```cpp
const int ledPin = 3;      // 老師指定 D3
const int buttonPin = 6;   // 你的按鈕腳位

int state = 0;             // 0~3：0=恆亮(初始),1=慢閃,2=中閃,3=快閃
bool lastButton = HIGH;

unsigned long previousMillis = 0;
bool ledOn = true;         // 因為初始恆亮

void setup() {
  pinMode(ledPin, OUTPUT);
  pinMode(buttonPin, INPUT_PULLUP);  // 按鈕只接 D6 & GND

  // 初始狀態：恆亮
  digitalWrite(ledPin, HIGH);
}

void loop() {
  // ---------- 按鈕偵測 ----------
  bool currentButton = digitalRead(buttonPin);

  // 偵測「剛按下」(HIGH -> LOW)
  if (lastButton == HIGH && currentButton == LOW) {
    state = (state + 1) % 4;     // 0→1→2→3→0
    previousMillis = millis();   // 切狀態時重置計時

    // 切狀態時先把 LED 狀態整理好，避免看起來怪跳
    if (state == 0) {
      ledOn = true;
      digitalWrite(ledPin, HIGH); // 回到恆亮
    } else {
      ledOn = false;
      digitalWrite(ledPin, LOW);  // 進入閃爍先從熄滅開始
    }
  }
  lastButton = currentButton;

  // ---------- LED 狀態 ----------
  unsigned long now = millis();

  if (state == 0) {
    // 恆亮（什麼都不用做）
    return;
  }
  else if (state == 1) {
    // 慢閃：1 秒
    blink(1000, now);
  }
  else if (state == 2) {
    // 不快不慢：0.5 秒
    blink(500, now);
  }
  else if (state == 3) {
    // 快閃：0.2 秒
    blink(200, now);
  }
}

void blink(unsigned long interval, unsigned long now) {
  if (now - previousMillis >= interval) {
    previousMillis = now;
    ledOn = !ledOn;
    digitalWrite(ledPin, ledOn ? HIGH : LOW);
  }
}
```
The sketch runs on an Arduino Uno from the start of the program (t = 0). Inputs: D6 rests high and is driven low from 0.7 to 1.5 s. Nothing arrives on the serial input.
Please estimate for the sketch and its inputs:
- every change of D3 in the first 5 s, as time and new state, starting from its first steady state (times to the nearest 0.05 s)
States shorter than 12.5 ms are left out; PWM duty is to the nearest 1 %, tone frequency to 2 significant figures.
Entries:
0 s high; 0.7 s low; 1.7 s high; 2.7 s low; 3.7 s high; 4.7 s low
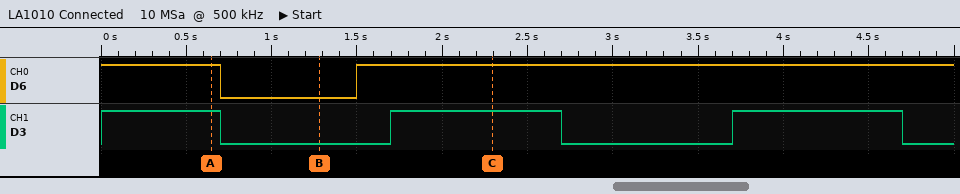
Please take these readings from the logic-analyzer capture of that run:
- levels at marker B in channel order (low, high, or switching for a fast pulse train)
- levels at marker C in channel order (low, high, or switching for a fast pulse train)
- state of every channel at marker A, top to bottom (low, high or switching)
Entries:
D6 low, D3 low
D6 high, D3 high
D6 high, D3 high
